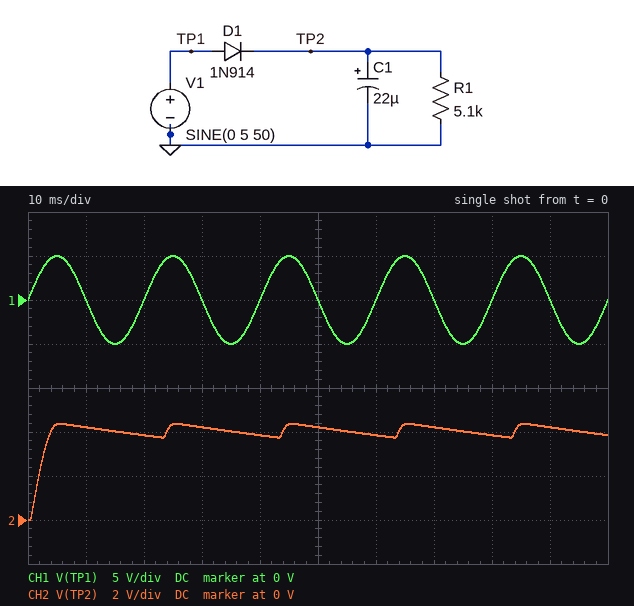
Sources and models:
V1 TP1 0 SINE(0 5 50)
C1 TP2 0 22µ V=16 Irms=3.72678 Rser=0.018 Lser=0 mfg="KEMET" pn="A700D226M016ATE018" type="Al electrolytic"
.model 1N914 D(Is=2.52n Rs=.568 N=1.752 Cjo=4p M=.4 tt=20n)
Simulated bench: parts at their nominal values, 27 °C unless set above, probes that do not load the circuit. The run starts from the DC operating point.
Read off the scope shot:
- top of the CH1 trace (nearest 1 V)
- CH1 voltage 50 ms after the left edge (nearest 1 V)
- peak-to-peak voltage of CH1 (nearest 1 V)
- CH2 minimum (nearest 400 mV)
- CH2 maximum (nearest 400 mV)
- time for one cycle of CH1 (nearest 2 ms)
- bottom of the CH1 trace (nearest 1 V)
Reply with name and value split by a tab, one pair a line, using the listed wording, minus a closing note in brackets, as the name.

top of the CH1 trace	5 V
CH1 voltage 50 ms after the left edge	0 V
peak-to-peak voltage of CH1	10 V
CH2 minimum	0 V
CH2 maximum	4.4 V
time for one cycle of CH1	20 ms
bottom of the CH1 trace	-5 V
